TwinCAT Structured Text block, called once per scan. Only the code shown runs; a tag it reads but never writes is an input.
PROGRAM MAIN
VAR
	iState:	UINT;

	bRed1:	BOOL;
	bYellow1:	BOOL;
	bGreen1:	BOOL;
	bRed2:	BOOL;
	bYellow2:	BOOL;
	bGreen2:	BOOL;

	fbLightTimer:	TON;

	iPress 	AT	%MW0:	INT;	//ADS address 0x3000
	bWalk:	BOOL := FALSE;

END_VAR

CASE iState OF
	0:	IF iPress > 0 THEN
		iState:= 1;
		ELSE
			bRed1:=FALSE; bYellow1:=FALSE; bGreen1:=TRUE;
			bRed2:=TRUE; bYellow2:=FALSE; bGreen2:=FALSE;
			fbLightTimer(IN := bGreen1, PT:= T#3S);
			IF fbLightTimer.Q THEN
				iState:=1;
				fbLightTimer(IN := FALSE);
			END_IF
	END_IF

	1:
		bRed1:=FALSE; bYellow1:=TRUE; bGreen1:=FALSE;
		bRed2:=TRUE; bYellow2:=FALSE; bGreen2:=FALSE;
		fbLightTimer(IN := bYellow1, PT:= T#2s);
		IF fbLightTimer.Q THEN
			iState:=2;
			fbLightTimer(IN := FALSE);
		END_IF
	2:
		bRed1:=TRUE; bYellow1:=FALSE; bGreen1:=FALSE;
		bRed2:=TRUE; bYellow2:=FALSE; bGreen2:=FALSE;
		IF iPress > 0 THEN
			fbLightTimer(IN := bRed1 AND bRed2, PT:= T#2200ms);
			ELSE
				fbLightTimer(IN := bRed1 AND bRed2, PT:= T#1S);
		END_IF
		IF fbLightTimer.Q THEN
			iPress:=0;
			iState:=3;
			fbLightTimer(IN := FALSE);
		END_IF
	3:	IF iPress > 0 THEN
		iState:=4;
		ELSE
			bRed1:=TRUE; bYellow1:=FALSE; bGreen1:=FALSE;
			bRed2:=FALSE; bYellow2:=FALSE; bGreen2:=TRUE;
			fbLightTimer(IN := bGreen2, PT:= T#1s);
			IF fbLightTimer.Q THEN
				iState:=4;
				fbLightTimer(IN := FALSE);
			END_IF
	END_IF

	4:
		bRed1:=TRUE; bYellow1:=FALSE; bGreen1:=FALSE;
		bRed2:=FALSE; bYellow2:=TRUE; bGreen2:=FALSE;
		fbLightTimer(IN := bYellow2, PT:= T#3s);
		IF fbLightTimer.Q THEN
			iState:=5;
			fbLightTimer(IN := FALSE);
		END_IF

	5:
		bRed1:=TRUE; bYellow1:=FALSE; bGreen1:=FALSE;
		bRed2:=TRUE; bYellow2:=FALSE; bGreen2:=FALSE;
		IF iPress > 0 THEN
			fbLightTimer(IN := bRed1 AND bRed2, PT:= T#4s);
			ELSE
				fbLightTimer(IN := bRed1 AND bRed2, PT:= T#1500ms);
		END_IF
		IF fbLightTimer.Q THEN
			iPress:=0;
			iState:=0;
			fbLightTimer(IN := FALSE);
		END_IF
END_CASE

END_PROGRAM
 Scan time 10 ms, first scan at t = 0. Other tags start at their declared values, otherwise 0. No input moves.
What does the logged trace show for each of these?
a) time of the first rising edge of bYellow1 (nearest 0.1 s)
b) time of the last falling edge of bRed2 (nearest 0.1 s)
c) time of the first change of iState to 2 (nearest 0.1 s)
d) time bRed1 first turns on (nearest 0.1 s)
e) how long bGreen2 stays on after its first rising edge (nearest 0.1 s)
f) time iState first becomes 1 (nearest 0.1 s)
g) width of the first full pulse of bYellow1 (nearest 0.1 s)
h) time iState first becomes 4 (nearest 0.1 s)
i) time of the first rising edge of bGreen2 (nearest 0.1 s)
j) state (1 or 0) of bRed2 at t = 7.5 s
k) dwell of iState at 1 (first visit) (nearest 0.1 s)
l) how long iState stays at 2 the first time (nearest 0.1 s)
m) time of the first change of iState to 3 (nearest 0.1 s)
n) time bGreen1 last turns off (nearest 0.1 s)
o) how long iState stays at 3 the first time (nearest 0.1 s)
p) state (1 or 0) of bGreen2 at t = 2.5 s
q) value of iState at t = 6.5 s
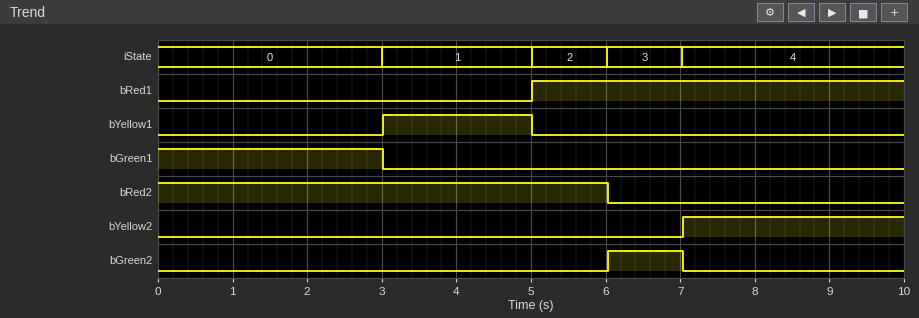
3.0 s
6.0 s
5.0 s
5.0 s
1.0 s
3.0 s
2.0 s
7.0 s
6.0 s
0
2.0 s
1.0 s
6.0 s
3.0 s
1.0 s
0
3
